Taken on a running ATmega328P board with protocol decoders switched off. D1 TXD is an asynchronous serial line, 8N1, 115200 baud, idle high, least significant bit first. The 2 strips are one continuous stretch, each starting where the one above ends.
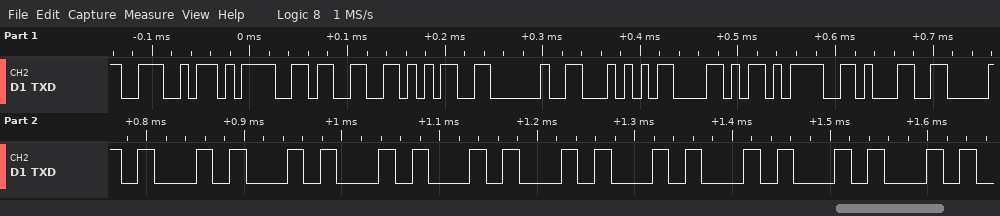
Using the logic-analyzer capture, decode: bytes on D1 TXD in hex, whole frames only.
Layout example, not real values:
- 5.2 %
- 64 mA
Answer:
- 0x4E 0x3D 0x33 0x35 0x20 0x54 0x58 0x3D 0x31 0x30 0x30 0x30 0x30 0x30 0x30 0x30 0x30 0x30 0x30
